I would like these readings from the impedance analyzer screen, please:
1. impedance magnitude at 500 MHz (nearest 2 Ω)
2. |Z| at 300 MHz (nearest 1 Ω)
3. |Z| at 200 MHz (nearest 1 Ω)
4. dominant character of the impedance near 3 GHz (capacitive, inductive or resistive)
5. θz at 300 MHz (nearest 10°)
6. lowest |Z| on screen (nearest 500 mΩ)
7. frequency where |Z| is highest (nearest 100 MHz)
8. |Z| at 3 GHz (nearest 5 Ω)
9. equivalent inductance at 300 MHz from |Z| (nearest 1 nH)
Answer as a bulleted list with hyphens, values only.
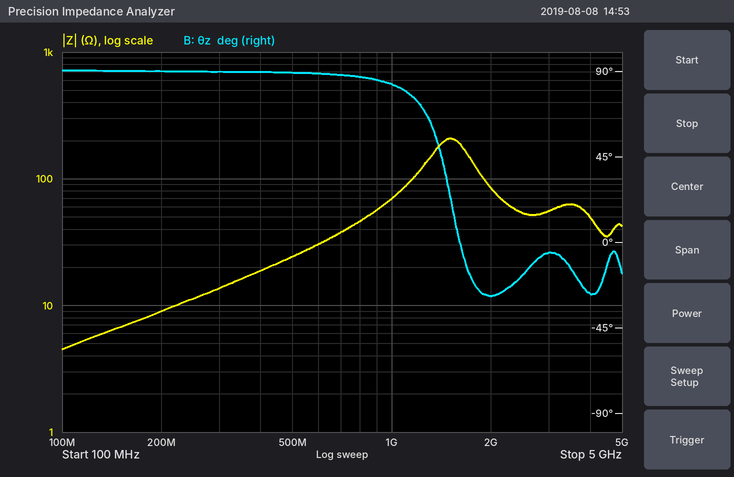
- 24 Ω
- 14 Ω
- 9 Ω
- resistive
- 90°
- 4.5 Ω
- 1.5 GHz
- 55 Ω
- 7 nH
